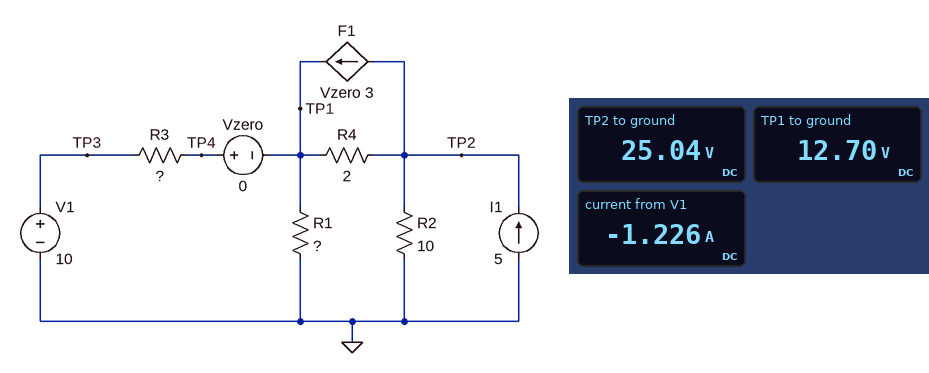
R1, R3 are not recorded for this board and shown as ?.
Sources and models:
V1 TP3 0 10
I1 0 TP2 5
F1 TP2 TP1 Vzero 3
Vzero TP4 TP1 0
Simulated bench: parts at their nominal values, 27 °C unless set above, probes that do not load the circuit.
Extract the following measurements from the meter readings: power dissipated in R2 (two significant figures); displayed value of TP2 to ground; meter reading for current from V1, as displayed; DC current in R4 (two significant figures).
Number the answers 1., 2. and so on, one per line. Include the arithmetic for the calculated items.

1. (25.04 V)^2 / 10 Ω = 63 W
2. 25.04 V
3. -1.226 A
4. (25.04 V - 12.7 V) / 2 Ω = 6.2 A
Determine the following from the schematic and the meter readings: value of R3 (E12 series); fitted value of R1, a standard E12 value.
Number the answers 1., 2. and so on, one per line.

1. 2.2 Ω
2. 10 Ω
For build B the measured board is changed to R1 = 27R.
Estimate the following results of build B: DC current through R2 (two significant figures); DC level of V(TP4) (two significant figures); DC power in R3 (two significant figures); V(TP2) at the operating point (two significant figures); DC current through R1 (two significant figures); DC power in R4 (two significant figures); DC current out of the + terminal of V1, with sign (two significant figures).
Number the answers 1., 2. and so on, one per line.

1. 2.8 A
2. 14 V
3. 6.2 W
4. 28 V
5. 510 mA
6. 100 W
7. -1.7 A
